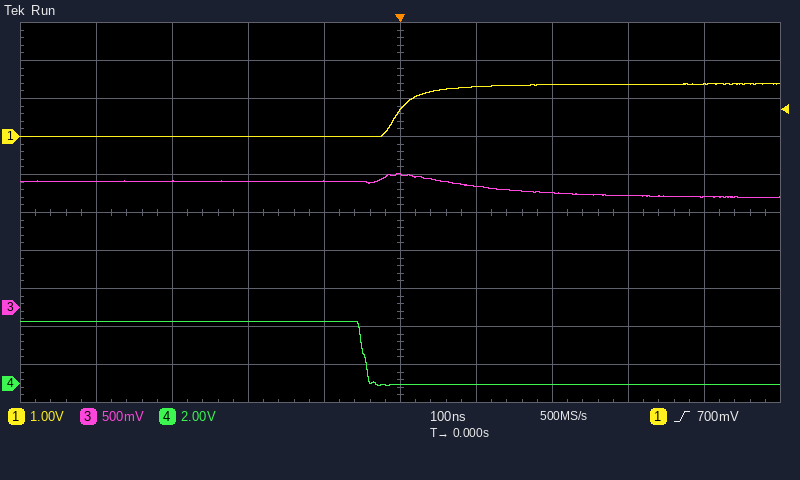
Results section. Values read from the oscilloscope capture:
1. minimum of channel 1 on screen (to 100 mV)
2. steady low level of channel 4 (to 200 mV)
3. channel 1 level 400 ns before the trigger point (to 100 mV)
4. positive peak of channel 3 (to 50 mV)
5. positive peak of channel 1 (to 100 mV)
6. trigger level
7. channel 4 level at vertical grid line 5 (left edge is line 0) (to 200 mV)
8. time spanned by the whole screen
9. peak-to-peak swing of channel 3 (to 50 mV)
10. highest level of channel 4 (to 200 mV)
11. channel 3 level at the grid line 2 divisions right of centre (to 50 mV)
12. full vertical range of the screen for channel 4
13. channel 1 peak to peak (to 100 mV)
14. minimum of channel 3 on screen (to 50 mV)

0.0 V
0.0 V
0.0 V
1.75 V
1.4 V
700 mV
0.0 V
1 µs
300 mV
3.2 V
1.50 V
20 V
1.4 V
1.45 V
